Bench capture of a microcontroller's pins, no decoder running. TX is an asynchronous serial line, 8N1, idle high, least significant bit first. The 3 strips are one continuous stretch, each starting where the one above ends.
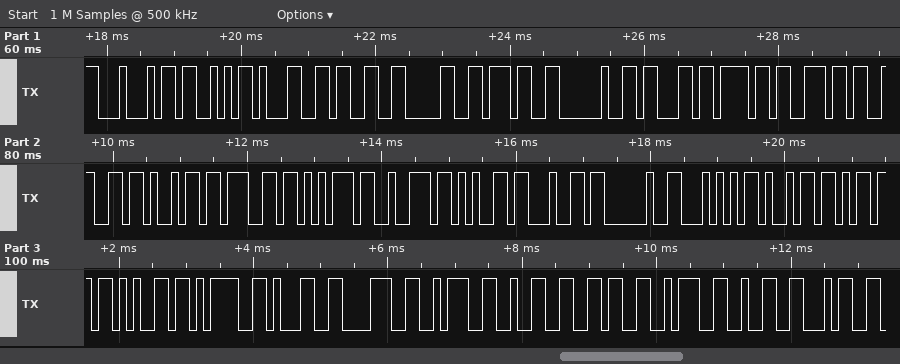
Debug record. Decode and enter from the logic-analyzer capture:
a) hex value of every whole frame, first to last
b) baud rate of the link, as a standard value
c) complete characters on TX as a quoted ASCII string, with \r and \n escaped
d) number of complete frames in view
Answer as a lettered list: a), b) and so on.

a) 44 53 31 33 30 37 20 63 6F 6E 66 69 67 75 72 65 64 20 54 69 6D 65 3D 31 38 3A 32 36 3A 32 34
b) 9600 baud
c) "DS1307 configured Time=18:26:24"
d) 31
